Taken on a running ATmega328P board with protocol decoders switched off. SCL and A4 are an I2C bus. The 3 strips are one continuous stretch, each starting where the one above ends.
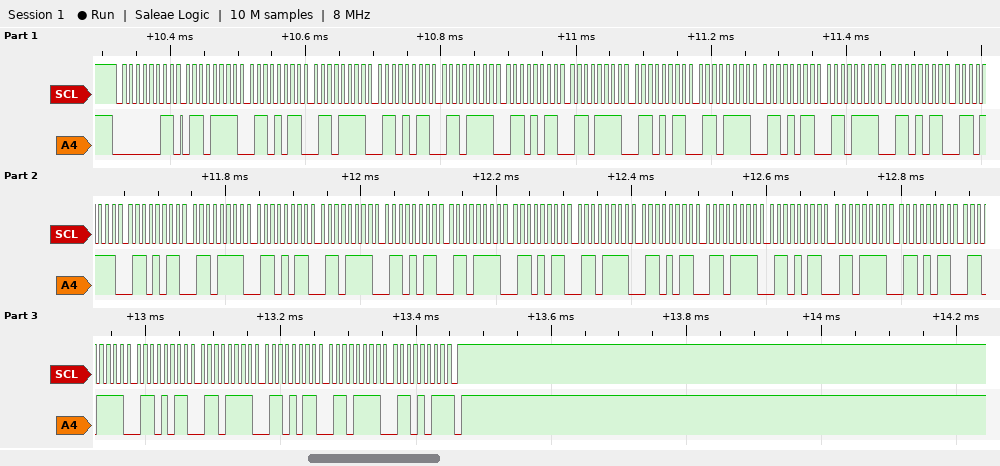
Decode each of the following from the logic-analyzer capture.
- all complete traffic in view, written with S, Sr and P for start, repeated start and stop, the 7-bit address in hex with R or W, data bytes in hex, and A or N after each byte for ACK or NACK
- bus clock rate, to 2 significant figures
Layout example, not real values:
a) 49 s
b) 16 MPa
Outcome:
a) S 01R A 6F A 6B A 6F A 6B A 6F A 6B A 6F A 6B A 6F A 6B A 6F A 6B A 6F A 6B A 6F A 6B A 6F A 6B A 6F A 6B A 6F A 6B A 6F A 6B A 6F A 6B A 6F A 6B A 6F A 6B A 6F A 6B N P
b) 100 kHz
